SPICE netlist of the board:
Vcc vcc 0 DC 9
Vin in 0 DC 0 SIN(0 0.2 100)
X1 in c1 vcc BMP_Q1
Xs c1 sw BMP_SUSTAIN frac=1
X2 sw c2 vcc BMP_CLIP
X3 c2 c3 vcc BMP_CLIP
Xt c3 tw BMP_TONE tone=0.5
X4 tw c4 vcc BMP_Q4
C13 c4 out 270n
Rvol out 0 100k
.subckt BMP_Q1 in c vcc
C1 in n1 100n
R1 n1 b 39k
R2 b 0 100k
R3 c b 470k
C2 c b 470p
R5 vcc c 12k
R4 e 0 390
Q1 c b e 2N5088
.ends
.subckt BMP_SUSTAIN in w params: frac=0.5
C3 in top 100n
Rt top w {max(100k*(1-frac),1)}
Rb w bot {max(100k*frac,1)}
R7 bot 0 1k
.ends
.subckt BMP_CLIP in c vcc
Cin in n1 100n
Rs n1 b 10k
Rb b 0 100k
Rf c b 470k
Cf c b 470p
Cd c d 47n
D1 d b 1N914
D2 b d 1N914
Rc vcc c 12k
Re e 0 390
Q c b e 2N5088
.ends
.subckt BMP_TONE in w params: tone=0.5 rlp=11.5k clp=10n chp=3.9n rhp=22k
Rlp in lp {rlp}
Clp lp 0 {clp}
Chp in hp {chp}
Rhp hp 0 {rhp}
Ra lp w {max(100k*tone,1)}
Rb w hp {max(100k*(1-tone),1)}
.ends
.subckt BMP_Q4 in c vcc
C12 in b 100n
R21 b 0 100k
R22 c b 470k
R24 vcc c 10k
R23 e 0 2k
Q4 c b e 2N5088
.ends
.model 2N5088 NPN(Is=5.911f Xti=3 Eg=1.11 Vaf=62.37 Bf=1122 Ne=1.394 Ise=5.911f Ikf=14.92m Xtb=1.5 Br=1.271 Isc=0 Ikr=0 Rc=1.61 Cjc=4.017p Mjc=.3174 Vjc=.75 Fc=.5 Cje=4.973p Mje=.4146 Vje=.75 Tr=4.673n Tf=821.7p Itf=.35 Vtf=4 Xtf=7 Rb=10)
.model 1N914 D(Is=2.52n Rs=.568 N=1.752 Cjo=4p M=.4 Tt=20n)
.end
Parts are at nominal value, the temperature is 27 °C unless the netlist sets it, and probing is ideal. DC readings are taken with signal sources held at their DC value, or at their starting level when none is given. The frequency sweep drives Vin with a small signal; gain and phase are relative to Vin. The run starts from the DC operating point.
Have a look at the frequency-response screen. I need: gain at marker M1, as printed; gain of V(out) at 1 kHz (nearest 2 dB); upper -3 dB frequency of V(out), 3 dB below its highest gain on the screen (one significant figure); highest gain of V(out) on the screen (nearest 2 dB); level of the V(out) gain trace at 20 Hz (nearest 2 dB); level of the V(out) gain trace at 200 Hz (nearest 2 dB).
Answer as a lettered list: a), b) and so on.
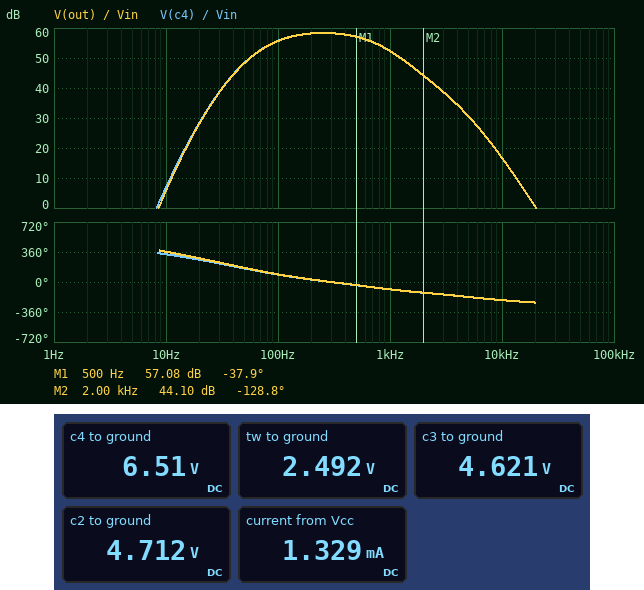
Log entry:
a) 57.08 dB
b) 52 dB
c) 700 Hz
d) 58 dB
e) 28 dB
f) 58 dB
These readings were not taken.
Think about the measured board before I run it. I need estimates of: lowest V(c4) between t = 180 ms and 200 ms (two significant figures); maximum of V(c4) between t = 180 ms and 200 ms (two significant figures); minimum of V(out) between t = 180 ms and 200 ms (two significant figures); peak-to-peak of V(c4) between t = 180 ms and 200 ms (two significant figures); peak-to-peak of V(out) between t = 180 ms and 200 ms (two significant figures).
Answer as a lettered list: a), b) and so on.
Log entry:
a) 3.8 V
b) 8.6 V
c) -2.6 V
d) 4.8 V
e) 4.7 V
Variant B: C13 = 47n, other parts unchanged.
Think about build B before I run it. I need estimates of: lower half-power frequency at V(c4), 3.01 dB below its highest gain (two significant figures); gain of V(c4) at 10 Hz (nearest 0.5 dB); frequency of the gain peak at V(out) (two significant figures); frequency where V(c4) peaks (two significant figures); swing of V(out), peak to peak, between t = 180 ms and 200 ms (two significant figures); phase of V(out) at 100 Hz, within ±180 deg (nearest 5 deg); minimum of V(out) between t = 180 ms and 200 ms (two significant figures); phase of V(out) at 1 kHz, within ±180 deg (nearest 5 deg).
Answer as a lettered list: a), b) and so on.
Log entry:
a) 94 Hz
b) 7.5 dB
c) 260 Hz
d) 250 Hz
e) 4.4 V
f) 105 deg
g) -2.3 V
h) -85 deg
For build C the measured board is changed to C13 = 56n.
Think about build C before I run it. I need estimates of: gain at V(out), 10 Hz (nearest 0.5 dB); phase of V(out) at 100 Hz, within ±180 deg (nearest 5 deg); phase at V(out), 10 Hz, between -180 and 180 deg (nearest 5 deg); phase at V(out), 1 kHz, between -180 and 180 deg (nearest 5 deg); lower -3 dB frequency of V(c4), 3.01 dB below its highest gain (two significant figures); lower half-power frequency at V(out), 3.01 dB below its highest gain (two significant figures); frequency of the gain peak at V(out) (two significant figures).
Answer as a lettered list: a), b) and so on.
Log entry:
a) -2.5 dB
b) 105 deg
c) 45 deg
d) -85 deg
e) 94 Hz
f) 98 Hz
g) 260 Hz
